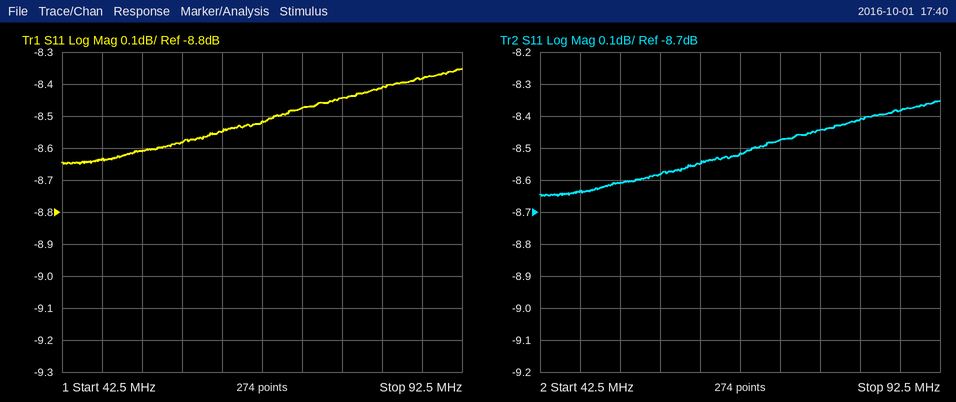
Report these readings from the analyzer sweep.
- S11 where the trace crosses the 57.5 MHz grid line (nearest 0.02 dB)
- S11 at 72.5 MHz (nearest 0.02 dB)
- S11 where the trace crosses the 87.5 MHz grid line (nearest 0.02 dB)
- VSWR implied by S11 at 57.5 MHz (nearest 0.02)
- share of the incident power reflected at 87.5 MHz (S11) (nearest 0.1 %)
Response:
-8.58 dB
-8.48 dB
-8.38 dB
2.18
14.5 %
